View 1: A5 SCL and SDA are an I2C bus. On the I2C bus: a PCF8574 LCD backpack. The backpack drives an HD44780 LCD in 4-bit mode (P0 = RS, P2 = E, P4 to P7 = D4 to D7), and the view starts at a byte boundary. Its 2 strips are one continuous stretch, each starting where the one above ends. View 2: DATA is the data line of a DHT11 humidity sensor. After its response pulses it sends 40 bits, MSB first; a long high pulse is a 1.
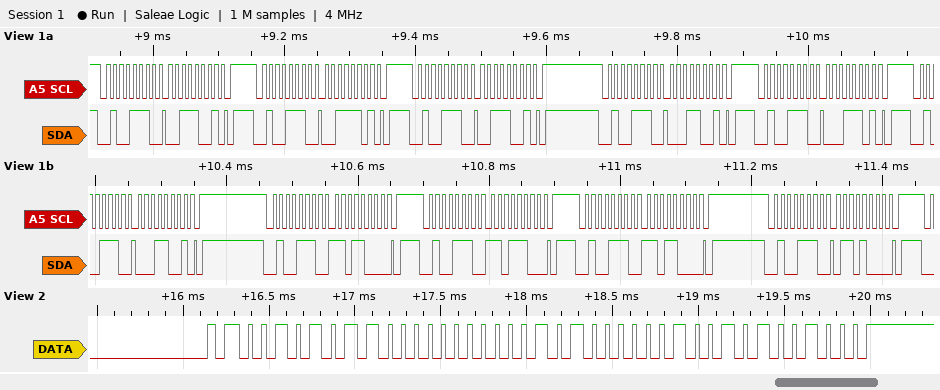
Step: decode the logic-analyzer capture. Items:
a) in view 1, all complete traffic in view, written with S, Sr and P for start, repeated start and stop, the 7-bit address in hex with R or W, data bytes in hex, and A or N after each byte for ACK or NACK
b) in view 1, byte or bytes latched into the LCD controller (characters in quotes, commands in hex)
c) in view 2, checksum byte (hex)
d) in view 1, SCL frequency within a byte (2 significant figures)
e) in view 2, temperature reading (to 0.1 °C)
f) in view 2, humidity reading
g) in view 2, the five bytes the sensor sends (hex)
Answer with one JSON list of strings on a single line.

["S 27W A 39 A P S 27W A 3D A P S 27W A 39 A P S 27W A 19 A P S 27W A 1D A P S 27W A 19 A P S 27W A D8 A P S 27W A DC A P S 27W A D8 A P S 27W A 68 A P", "'1'", "0x48", "100 kHz", "20.9 °C", "43 %", "2B 00 14 09 48"]
